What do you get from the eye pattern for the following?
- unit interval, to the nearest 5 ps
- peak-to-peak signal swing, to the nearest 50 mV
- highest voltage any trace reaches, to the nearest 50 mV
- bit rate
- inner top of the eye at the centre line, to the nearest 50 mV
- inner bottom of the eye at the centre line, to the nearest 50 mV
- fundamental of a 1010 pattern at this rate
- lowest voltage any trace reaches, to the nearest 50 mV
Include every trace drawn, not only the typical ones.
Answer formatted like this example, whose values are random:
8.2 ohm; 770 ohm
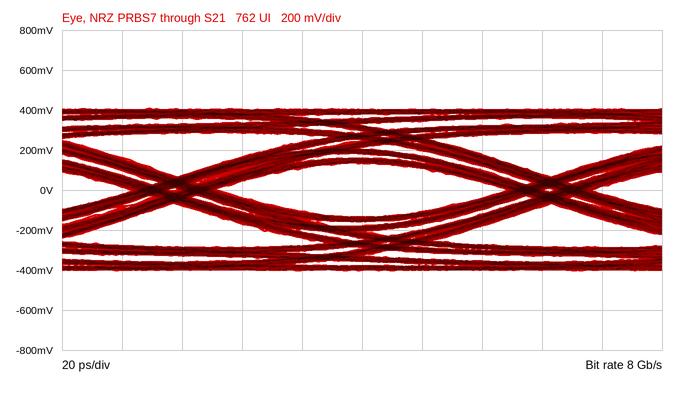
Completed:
125 ps; 800 mV; 400 mV; 8 Gb/s; 150 mV; -150 mV; 4 GHz; -400 mV
